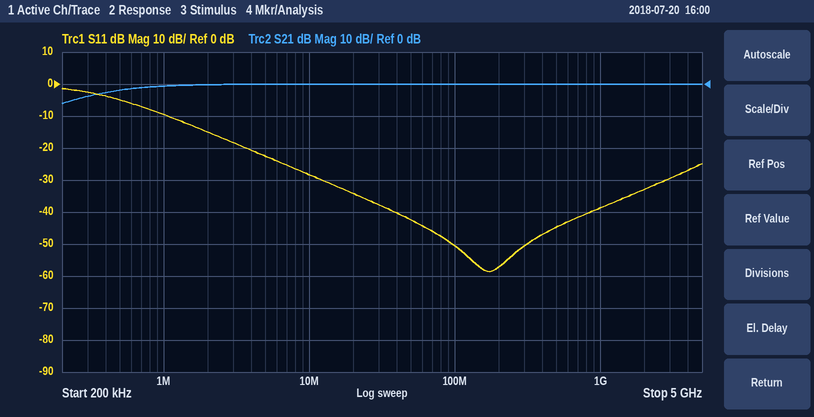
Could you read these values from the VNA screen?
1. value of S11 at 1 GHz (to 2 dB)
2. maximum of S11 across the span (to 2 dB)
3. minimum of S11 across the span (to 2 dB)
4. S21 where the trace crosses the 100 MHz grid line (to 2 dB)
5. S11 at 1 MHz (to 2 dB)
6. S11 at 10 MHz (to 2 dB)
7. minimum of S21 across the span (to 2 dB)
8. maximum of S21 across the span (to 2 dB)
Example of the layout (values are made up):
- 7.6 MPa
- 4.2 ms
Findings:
- -38 dB
- -2 dB
- -58 dB
- 0 dB
- -10 dB
- -28 dB
- -6 dB
- 0 dB
